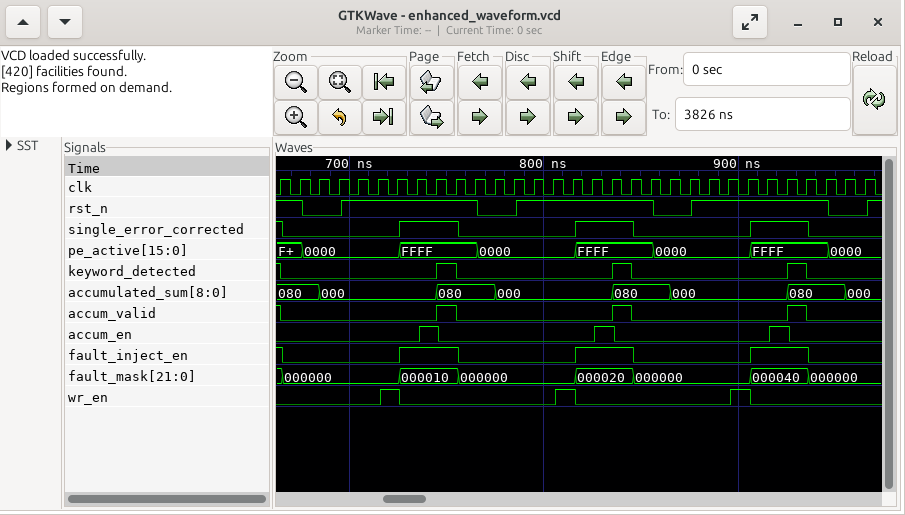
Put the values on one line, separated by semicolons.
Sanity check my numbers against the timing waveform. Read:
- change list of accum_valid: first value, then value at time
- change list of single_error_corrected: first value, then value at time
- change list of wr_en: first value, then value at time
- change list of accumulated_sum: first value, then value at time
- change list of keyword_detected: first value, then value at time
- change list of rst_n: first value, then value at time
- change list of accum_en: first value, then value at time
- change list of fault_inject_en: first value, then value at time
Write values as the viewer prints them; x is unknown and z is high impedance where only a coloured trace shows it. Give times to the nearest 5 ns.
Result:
1, 0 at 665 ns, 1 at 745 ns, 0 at 755 ns, 1 at 835 ns, 0 at 845 ns, 1 at 925 ns, 0 at 935 ns; 1, 0 at 665 ns, 1 at 725 ns, 0 at 755 ns, 1 at 815 ns, 0 at 845 ns, 1 at 905 ns, 0 at 935 ns; 0, 1 at 715 ns, 0 at 725 ns, 1 at 805 ns, 0 at 815 ns, 1 at 895 ns, 0 at 905 ns; 080, 000 at 685 ns, 080 at 745 ns, 000 at 775 ns, 080 at 835 ns, 000 at 865 ns, 080 at 925 ns, 000 at 955 ns; 1, 0 at 665 ns, 1 at 745 ns, 0 at 755 ns, 1 at 835 ns, 0 at 845 ns, 1 at 925 ns, 0 at 935 ns; 1, 0 at 675 ns, 1 at 695 ns, 0 at 765 ns, 1 at 785 ns, 0 at 855 ns, 1 at 875 ns, 0 at 945 ns, 1 at 965 ns; 0, 1 at 735 ns, 0 at 745 ns, 1 at 825 ns, 0 at 835 ns, 1 at 915 ns, 0 at 925 ns; 1, 0 at 665 ns, 1 at 725 ns, 0 at 755 ns, 1 at 815 ns, 0 at 845 ns, 1 at 905 ns, 0 at 935 ns
